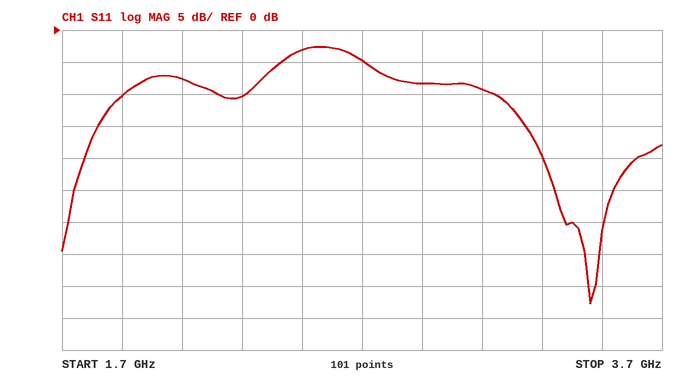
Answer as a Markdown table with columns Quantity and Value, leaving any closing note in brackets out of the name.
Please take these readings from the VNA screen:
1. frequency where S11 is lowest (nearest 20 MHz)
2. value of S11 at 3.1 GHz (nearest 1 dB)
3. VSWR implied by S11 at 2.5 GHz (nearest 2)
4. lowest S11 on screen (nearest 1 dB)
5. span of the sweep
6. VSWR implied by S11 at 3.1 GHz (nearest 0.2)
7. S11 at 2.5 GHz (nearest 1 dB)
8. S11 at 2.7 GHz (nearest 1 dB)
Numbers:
| Quantity | Value |
|---|---|
| frequency where S11 is lowest | 3.46 GHz |
| value of S11 at 3.1 GHz | -9 dB |
| VSWR implied by S11 at 2.5 GHz | 6 |
| lowest S11 on screen | -43 dB |
| span of the sweep | 2 GHz |
| VSWR implied by S11 at 3.1 GHz | 2.0 |
| S11 at 2.5 GHz | -3 dB |
| S11 at 2.7 GHz | -5 dB |
